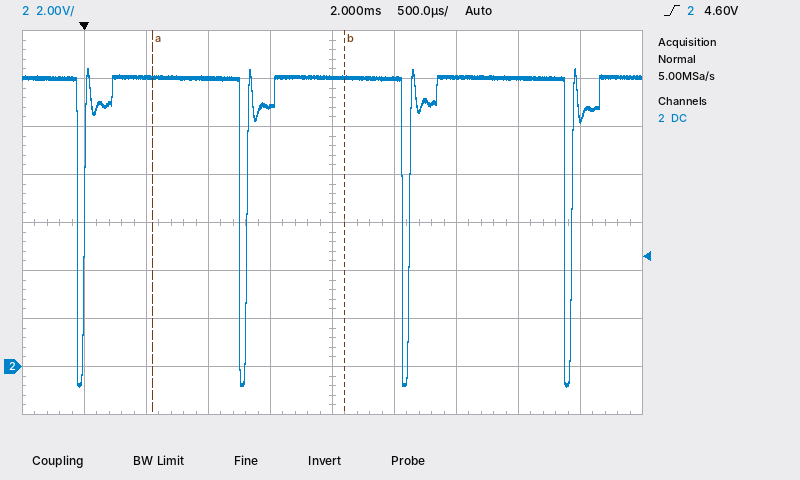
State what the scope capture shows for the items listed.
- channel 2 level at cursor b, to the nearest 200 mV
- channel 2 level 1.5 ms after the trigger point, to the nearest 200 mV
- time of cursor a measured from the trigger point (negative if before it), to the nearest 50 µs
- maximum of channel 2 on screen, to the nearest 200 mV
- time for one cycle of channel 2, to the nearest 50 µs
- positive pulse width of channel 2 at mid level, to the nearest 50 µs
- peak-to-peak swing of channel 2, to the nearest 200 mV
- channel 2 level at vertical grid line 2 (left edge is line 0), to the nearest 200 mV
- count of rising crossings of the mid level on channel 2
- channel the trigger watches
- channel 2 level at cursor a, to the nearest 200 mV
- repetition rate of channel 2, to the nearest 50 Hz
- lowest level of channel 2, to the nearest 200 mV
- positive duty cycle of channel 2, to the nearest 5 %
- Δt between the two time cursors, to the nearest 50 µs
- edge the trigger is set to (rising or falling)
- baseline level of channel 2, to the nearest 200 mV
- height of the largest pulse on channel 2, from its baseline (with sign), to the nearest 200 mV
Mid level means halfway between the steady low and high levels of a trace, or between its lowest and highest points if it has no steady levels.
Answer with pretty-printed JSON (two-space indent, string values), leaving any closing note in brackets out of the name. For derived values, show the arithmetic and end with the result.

{
  "channel 2 level at cursor b, to the nearest 200 mV": "12.0 V",
  "channel 2 level 1.5 ms after the trigger point, to the nearest 200 mV": "10.8 V",
  "time of cursor a measured from the trigger point (negative if before it), to the nearest 50 µs": "+550 µs",
  "maximum of channel 2 on screen, to the nearest 200 mV": "12.4 V",
  "time for one cycle of channel 2, to the nearest 50 µs": "1.30 ms",
  "positive pulse width of channel 2 at mid level, to the nearest 50 µs": "1.25 ms",
  "peak-to-peak swing of channel 2, to the nearest 200 mV": "12.4 V − (-800 mV) = 13.2 V",
  "channel 2 level at vertical grid line 2 (left edge is line 0), to the nearest 200 mV": "12.0 V",
  "count of rising crossings of the mid level on channel 2": "4",
  "channel the trigger watches": "channel 2",
  "channel 2 level at cursor a, to the nearest 200 mV": "12.0 V",
  "repetition rate of channel 2, to the nearest 50 Hz": "1 / 1.30 ms ≈ 769 Hz, so 750 Hz to the nearest 50 Hz",
  "lowest level of channel 2, to the nearest 200 mV": "-800 mV",
  "positive duty cycle of channel 2, to the nearest 5 %": "1.25 ms / 1.30 ms ≈ 96.2 %, so 95 % to the nearest 5 %",
  "Δt between the two time cursors, to the nearest 50 µs": "1.55 ms",
  "edge the trigger is set to": "rising",
  "baseline level of channel 2, to the nearest 200 mV": "12.0 V",
  "height of the largest pulse on channel 2, from its baseline (with sign), to the nearest 200 mV": "-800 mV − (12.0 V) = -12.8 V"
}
